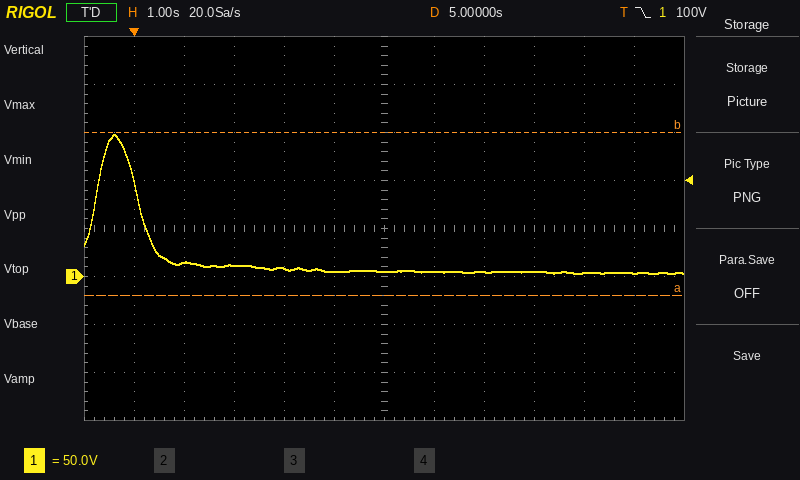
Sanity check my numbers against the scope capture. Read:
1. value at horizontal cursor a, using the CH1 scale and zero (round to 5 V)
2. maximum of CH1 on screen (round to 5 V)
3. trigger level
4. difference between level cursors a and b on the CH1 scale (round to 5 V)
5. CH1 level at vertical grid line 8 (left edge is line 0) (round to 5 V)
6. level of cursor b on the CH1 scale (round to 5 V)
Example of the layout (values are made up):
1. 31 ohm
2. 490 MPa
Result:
1. -20 V
2. 150 V
3. 100 V
4. 170 V
5. 5 V
6. 150 V
